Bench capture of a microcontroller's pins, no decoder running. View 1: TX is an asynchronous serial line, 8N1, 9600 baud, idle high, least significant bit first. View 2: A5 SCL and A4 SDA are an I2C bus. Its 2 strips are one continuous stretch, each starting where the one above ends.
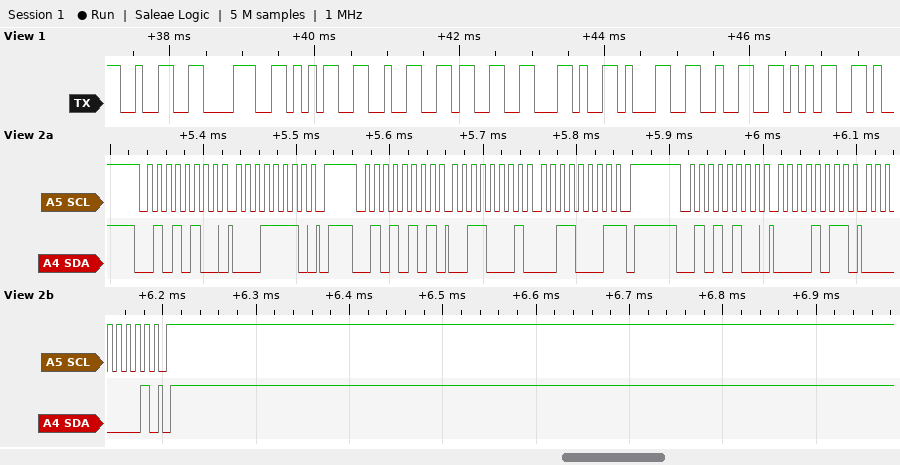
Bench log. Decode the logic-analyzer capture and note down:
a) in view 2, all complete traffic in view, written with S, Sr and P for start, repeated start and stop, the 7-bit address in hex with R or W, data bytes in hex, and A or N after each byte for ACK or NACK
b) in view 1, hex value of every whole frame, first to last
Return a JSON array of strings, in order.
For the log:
["S 2AW A 1E A P S 2AR A 31 A 31 N P S 2AW A 0B A 01 A P", "32 38 35 32 33 2C 31 32 35"]
